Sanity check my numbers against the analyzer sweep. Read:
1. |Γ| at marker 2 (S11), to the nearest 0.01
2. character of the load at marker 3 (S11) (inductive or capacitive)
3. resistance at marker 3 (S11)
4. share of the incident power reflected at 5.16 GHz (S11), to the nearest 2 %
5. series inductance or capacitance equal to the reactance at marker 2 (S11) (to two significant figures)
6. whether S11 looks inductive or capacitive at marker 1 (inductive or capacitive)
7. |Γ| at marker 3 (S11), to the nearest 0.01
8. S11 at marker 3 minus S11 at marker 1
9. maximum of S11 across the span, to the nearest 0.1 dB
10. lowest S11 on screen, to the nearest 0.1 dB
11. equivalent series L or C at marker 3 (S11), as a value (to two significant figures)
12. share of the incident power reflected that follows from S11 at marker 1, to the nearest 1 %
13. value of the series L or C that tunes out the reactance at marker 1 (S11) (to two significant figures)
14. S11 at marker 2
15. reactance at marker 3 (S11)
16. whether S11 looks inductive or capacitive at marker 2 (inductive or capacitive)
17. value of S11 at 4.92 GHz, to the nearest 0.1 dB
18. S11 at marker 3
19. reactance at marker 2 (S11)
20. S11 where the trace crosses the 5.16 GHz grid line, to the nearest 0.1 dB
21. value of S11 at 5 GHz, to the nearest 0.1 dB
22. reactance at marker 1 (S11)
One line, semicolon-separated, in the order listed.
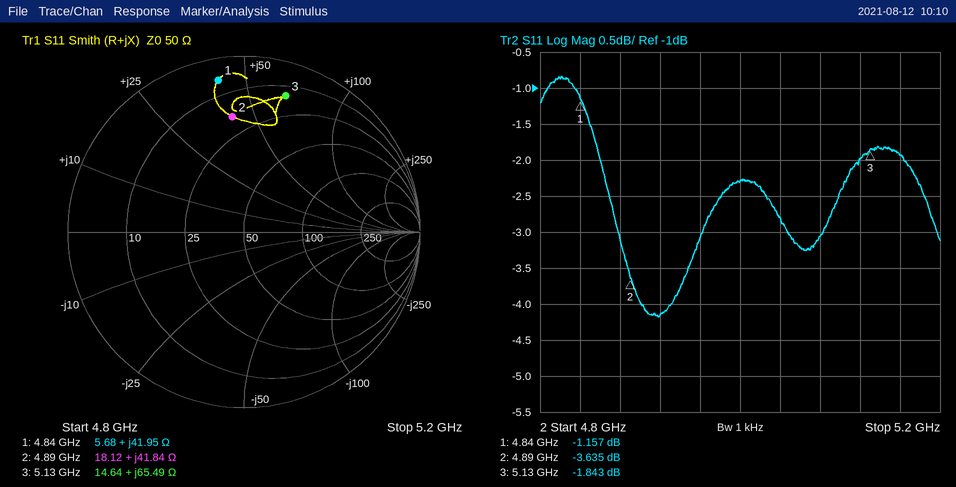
0.66; inductive; 14.64 Ω; 64 %; 1.4 nH; inductive; 0.81; -0.686 dB; -0.8 dB; -4.2 dB; 2.0 nH; 77 %; 780 fF; -3.635 dB; +65.49 Ω; inductive; -4.1 dB; -1.843 dB; +41.84 Ω; -1.9 dB; -2.3 dB; +41.95 Ω
